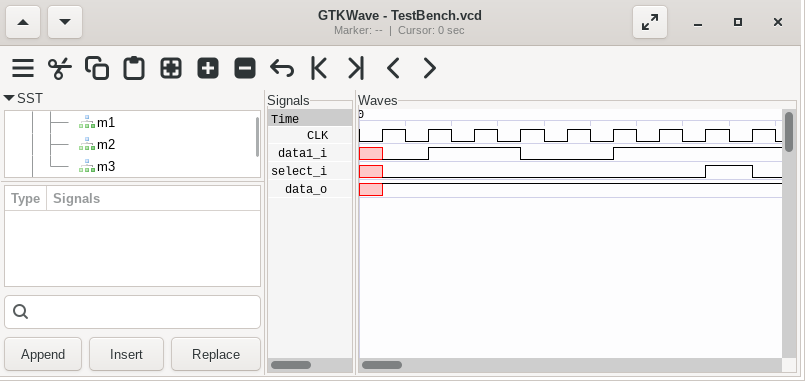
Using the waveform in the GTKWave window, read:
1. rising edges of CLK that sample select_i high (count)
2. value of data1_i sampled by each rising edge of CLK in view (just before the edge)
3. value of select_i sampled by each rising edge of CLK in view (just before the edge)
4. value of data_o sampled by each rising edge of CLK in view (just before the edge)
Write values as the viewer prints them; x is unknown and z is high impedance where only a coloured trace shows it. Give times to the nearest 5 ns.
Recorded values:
1
x 0 1 1 0 0 1 1 1
x 0 0 0 0 0 0 0 1
x 1 1 1 1 1 1 1 1
